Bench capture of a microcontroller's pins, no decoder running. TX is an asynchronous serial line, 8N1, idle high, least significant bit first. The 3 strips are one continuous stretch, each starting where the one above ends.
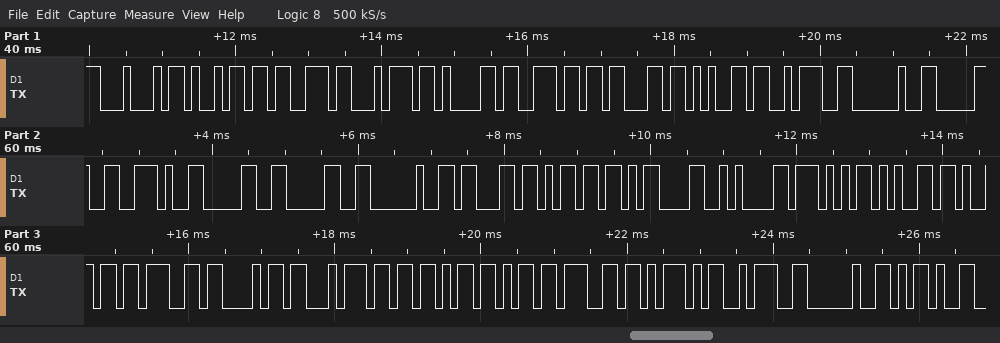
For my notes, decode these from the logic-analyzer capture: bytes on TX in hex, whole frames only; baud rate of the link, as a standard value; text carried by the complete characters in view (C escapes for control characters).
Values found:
44 69 73 74 61 6E 63 65 3A 20 30 2E 30 30 20 63 6D 0D 0A 57 65 69 67 68 74 5B 6B 67 5D 3A 20 2D
9600 baud
"Distance: 0.00 cm\r\nWeight[kg]: -"
